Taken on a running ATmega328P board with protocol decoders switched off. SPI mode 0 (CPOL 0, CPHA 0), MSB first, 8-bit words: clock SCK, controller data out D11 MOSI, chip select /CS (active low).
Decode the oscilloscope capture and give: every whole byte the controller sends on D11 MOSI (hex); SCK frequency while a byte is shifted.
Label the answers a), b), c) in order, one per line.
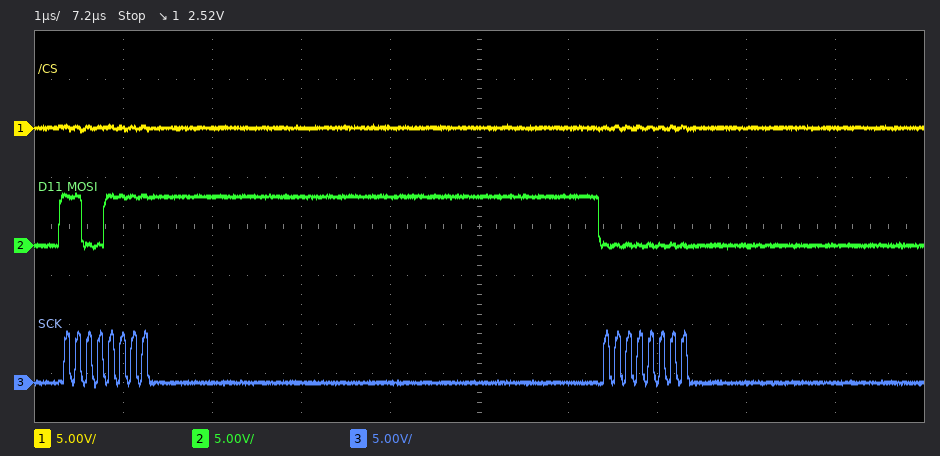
a) CF 00
b) 8 MHz
